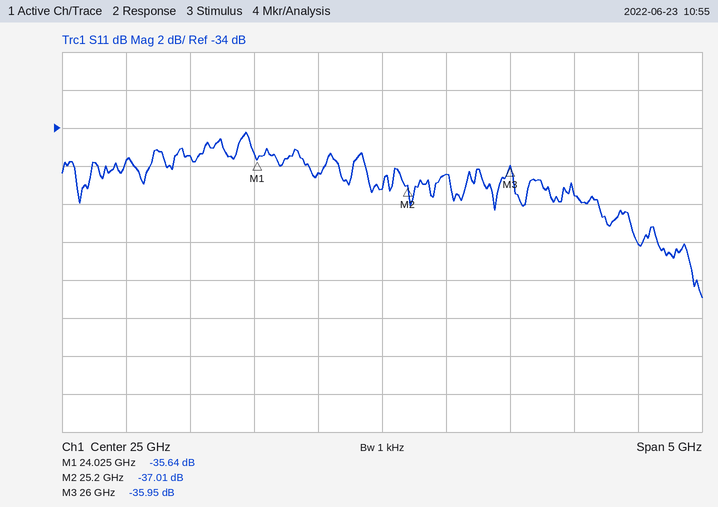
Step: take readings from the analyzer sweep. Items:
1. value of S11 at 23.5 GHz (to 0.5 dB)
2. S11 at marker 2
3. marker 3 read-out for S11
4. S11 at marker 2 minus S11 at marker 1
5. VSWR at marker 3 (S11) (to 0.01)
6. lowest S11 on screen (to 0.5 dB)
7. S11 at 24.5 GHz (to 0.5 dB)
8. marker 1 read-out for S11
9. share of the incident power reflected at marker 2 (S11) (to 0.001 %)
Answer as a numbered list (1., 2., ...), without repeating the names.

1. -35.5 dB
2. -37.01 dB
3. -35.95 dB
4. -1.37 dB
5. 1.03
6. -43.0 dB
7. -36.5 dB
8. -35.64 dB
9. 0.020 %
